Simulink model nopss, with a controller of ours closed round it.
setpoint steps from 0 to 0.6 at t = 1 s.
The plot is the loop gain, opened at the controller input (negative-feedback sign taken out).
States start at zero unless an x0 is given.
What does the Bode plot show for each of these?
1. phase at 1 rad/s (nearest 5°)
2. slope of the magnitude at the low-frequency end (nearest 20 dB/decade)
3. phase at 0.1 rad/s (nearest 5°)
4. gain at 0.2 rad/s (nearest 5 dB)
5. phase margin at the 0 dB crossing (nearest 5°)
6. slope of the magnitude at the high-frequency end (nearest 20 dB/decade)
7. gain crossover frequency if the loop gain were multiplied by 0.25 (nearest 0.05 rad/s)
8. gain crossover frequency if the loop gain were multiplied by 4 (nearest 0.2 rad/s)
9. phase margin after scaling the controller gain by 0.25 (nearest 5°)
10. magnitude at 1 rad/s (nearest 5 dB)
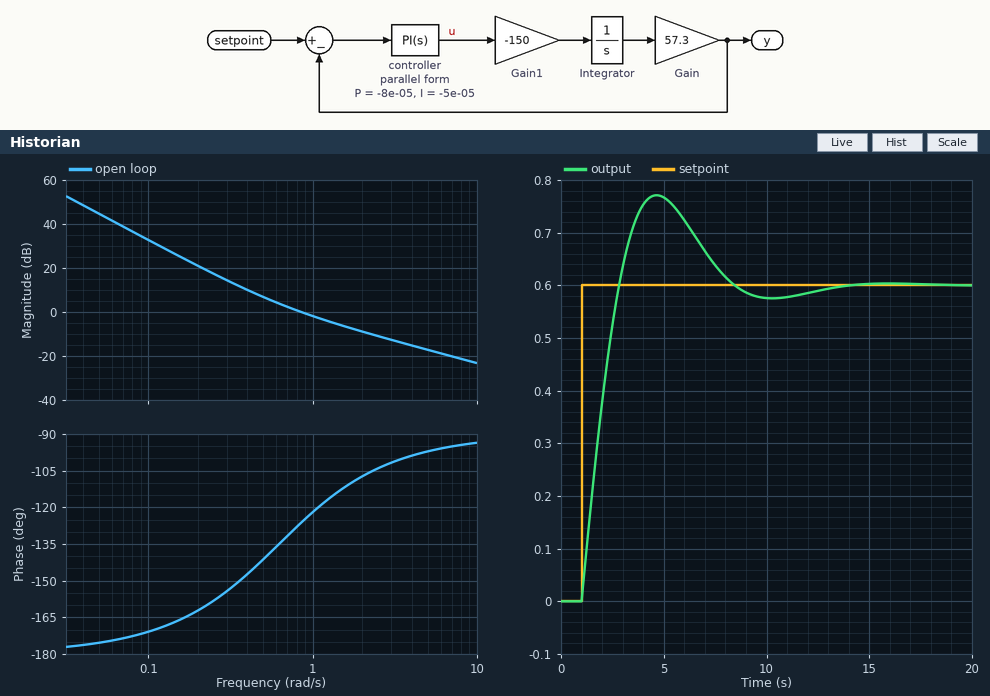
-120°
-40 dB/decade
-170°
20 dB
55°
-20 dB/decade
0.35 rad/s
2.8 rad/s
30°
0 dB
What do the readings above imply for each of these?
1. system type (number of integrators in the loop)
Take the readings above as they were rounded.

2
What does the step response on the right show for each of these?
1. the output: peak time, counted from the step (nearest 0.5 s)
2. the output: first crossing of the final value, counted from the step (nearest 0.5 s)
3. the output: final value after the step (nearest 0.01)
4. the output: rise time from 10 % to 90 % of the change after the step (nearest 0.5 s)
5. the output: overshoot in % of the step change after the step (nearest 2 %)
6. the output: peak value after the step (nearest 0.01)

3.5 s
2.0 s
0.60
1.5 s
28 %
0.77
